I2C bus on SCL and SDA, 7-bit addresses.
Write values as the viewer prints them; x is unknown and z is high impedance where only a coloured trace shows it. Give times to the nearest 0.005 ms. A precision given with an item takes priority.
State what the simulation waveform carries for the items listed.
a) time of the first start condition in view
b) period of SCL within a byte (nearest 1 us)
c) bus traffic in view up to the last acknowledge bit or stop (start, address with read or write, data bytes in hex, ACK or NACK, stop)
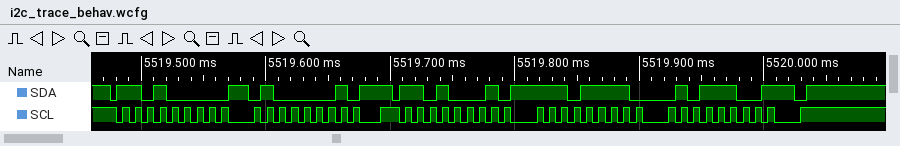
5519.475 ms
10 us
start, address 68 write ACK, 41 ACK, repeated start, address 68 read ACK, EF ACK, 5C NACK, stop
